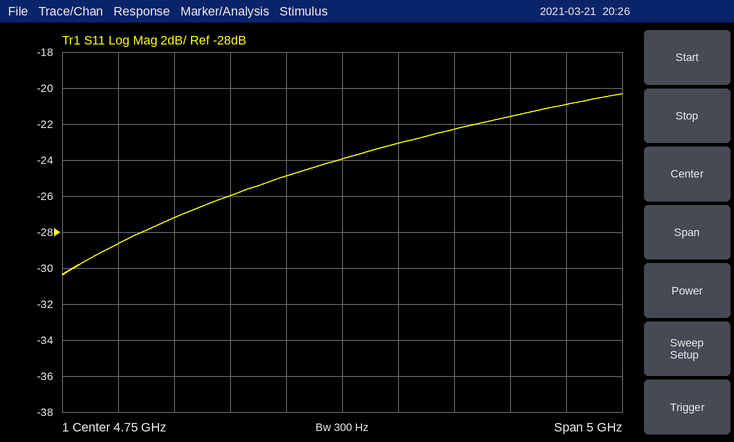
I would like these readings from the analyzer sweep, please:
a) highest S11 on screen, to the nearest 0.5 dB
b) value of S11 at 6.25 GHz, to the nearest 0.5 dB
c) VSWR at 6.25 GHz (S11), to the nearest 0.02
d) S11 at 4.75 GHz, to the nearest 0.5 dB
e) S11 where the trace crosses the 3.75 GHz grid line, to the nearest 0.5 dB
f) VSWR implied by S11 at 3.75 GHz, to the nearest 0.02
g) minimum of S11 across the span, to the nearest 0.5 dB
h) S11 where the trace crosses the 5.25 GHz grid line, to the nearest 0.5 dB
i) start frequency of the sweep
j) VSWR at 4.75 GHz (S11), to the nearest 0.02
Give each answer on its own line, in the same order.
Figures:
-20.5 dB
-21.5 dB
1.18
-24.0 dB
-26.0 dB
1.10
-30.5 dB
-23.0 dB
2.25 GHz
1.14
